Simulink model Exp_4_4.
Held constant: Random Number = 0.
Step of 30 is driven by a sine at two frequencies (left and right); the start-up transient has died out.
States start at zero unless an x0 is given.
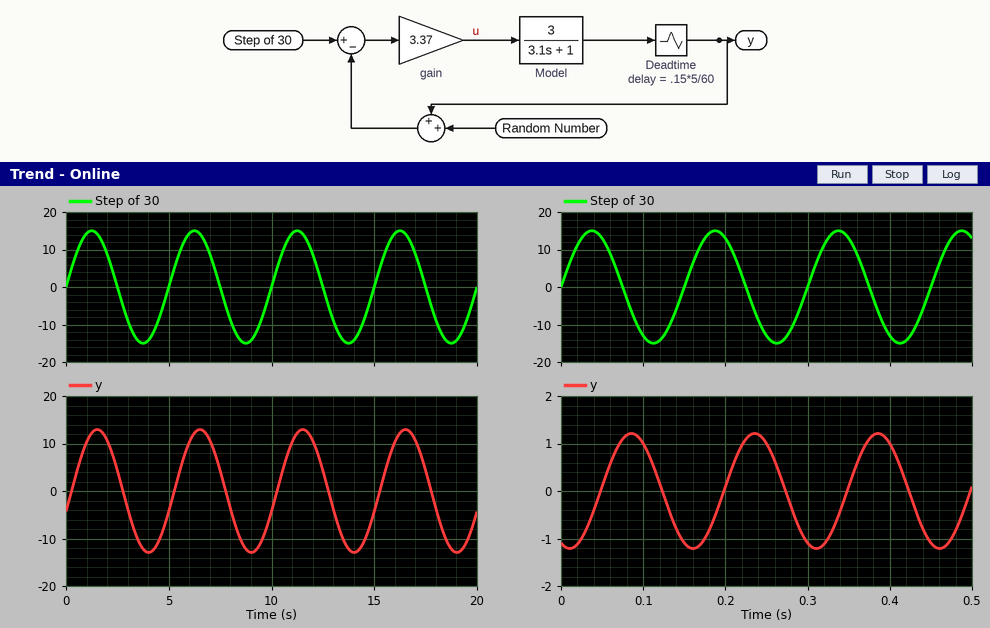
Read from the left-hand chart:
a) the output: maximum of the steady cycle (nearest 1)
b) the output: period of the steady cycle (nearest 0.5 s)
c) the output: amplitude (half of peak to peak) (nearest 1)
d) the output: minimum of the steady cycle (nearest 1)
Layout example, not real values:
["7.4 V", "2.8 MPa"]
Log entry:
["13", "5.0 s", "13", "-13"]
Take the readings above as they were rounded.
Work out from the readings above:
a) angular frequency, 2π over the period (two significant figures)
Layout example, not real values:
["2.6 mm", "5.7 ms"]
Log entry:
["1.3 rad/s"]
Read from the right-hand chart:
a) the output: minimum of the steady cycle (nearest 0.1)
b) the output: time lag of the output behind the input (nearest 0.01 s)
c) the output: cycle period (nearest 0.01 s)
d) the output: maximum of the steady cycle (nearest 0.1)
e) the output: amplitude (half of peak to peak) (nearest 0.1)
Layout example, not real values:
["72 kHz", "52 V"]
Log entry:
["-1.2", "0.05 s", "0.15 s", "1.2", "1.2"]
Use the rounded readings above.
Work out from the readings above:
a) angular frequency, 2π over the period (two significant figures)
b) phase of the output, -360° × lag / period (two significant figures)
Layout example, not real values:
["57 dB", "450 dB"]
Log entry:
["42 rad/s", "-120°"]
